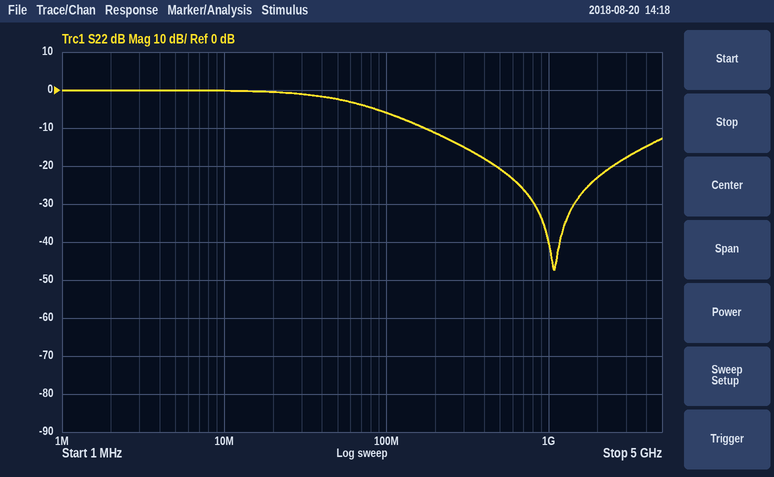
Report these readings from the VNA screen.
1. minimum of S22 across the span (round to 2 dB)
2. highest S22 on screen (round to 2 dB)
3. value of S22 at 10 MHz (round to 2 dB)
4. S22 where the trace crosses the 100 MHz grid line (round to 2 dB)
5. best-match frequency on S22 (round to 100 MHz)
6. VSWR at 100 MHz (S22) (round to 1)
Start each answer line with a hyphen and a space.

- -48 dB
- 0 dB
- 0 dB
- -6 dB
- 1.1 GHz
- 3
